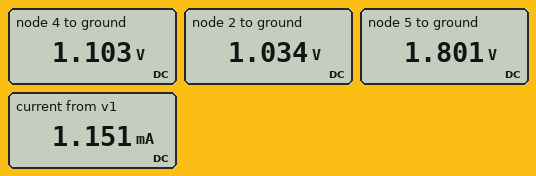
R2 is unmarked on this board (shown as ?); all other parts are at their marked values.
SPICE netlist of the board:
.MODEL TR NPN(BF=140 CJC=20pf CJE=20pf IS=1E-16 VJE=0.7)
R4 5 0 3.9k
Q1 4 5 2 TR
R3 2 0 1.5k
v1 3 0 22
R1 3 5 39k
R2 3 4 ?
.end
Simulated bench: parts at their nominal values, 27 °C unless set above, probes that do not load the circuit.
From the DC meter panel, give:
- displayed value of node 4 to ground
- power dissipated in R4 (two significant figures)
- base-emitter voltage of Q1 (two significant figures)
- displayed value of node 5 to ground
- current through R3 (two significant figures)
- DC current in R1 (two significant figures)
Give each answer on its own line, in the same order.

1.103 V
830 µW
770 mV
1.801 V
690 µA
520 µA
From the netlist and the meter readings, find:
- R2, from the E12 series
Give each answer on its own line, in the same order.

33 kΩ
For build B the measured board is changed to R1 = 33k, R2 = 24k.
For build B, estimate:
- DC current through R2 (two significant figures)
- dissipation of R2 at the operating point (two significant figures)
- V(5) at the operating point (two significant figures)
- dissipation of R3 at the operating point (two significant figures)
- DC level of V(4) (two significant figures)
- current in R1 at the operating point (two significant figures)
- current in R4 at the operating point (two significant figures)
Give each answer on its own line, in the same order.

860 µA
18 mW
2.1 V
1.2 mW
1.4 V
600 µA
550 µA
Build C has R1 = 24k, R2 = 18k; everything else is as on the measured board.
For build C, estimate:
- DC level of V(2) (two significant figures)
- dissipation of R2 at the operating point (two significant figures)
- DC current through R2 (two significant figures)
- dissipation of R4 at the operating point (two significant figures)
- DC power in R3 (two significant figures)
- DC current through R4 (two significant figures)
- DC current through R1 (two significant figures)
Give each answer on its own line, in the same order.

1.9 V
22 mW
1.1 mA
1.8 mW
2.3 mW
680 µA
810 µA
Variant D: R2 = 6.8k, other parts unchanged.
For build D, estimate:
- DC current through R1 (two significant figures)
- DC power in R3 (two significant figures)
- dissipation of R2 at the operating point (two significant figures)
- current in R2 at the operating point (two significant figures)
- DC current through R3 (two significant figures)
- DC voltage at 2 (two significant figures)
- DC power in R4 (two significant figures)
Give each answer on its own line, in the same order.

510 µA
980 µW
4.4 mW
800 µA
810 µA
1.2 V
1.0 mW
